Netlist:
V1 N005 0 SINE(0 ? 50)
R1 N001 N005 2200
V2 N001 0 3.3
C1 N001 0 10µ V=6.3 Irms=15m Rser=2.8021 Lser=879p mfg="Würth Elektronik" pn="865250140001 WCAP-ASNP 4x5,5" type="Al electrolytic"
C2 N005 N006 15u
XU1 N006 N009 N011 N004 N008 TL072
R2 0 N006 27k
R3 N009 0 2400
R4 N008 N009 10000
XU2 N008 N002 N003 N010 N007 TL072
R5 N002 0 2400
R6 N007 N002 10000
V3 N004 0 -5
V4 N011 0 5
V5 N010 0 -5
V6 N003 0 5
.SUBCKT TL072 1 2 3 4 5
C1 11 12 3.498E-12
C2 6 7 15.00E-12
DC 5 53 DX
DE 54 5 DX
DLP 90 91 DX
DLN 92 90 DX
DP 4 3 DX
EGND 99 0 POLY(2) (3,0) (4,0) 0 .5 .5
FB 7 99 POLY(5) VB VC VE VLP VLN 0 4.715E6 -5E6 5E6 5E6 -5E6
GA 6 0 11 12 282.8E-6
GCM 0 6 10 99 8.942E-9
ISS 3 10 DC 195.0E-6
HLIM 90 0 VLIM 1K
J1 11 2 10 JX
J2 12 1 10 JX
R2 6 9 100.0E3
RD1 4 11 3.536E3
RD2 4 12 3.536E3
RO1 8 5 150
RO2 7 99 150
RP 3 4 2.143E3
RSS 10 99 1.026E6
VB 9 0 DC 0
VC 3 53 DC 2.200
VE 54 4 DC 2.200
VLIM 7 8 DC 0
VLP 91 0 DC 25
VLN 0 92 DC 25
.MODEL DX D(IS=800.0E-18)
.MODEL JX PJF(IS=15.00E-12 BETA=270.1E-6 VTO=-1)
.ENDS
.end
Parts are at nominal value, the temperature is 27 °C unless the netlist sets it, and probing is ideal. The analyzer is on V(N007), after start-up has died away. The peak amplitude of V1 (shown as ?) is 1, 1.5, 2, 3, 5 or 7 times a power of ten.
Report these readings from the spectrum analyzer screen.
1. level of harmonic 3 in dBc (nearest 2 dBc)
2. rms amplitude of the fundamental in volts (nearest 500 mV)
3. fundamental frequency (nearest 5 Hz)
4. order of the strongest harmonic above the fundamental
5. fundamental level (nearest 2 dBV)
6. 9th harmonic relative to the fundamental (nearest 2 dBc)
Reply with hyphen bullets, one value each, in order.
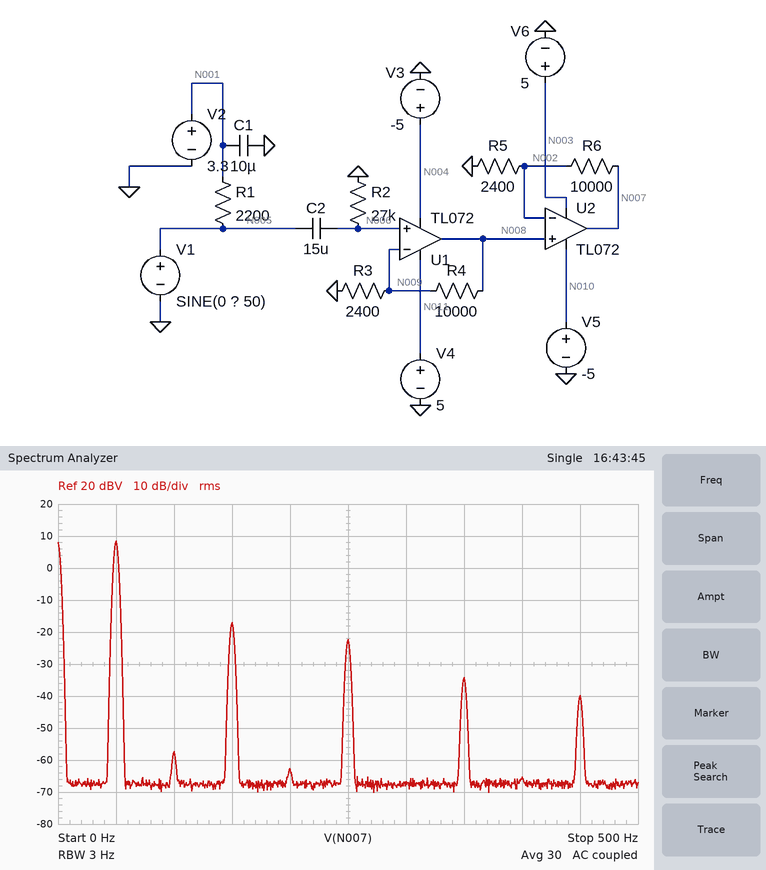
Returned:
- -26 dBc
- 2.5 V
- 50 Hz
- 3
- 8 dBV
- -48 dBc
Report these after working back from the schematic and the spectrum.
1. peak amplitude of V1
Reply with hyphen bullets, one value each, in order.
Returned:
- 150 mV
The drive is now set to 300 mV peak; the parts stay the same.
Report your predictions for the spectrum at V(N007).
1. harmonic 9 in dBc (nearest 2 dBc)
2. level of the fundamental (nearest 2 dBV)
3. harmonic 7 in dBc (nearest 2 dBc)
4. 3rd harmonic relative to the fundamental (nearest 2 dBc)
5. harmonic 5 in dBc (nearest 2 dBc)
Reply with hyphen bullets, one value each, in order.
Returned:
- -34 dBc
- 10 dBV
- -46 dBc
- -12 dBc
- -22 dBc
